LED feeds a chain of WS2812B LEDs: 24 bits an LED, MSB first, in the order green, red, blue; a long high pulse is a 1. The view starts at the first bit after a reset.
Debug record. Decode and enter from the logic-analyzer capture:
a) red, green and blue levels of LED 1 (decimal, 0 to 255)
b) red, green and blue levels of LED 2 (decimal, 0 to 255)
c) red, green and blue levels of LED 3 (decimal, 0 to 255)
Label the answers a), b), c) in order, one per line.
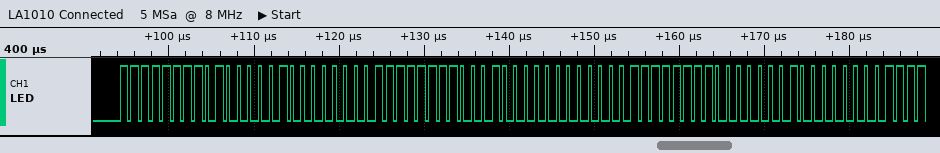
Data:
a) 65, 255, 0
b) 16, 255, 0
c) 1, 255, 0
